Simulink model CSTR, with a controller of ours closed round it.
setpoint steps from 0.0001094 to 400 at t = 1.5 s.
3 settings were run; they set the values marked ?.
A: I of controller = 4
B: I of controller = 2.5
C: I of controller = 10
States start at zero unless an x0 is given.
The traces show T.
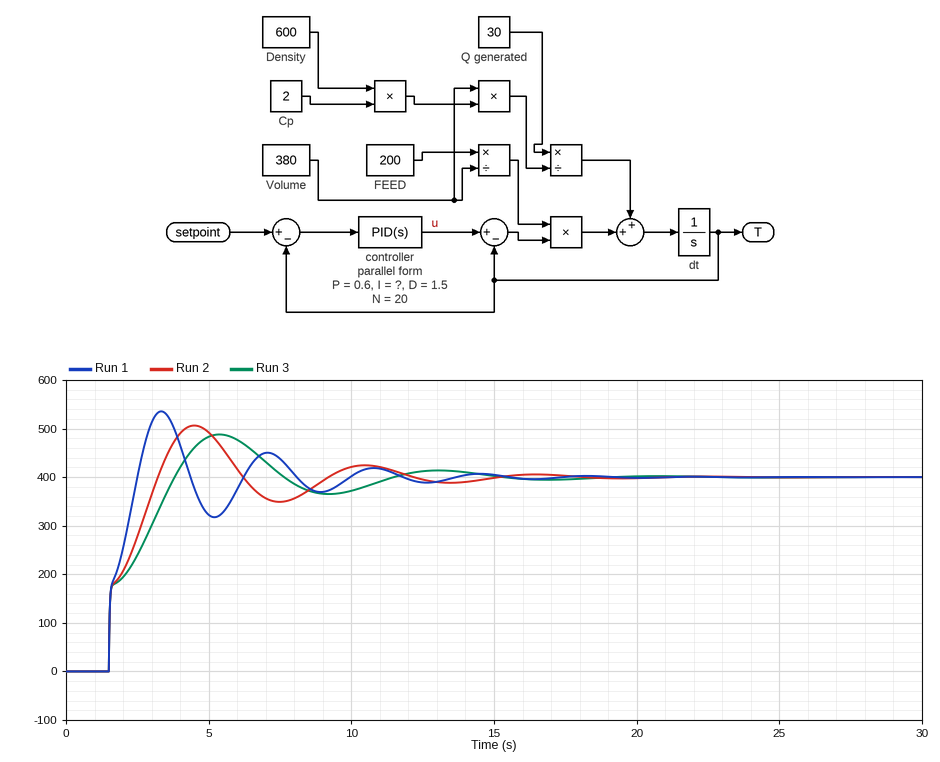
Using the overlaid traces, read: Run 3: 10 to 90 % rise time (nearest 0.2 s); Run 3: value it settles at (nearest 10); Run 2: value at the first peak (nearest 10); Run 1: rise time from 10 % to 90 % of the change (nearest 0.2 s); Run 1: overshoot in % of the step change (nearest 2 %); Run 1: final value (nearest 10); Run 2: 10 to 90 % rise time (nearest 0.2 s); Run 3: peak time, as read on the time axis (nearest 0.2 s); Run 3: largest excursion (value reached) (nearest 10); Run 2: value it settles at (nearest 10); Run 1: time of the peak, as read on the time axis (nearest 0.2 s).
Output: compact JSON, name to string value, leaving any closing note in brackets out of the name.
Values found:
{"Run 3: 10 to 90 % rise time": "2.0 s", "Run 3: value it settles at": "400", "Run 2: value at the first peak": "510", "Run 1: rise time from 10 % to 90 % of the change": "0.8 s", "Run 1: overshoot in % of the step change": "34 %", "Run 1: final value": "400", "Run 2: 10 to 90 % rise time": "1.4 s", "Run 3: peak time, as read on the time axis": "5.4 s", "Run 3: largest excursion (value reached)": "490", "Run 2: value it settles at": "400", "Run 1: time of the peak, as read on the time axis": "3.4 s"}
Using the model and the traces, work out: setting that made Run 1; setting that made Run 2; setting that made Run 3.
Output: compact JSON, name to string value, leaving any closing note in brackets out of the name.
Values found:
{"setting that made Run 1": "C", "setting that made Run 2": "A", "setting that made Run 3": "B"}
